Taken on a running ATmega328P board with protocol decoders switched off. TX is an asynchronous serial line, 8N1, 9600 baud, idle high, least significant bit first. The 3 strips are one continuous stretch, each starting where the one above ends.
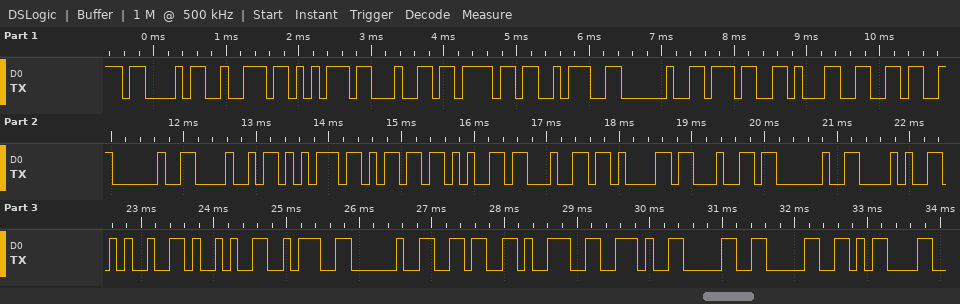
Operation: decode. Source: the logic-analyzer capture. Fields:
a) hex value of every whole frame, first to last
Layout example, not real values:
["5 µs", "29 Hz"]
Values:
["43 72 75 64 6F 3A 20 37 31 36 20 48 75 6D 65 64 61 64 20 28 25 29 3A 20 36 39 2E 30 30 0D"]
